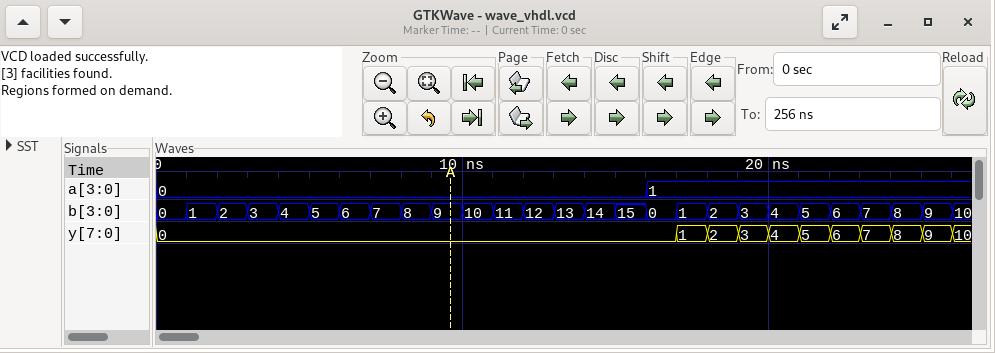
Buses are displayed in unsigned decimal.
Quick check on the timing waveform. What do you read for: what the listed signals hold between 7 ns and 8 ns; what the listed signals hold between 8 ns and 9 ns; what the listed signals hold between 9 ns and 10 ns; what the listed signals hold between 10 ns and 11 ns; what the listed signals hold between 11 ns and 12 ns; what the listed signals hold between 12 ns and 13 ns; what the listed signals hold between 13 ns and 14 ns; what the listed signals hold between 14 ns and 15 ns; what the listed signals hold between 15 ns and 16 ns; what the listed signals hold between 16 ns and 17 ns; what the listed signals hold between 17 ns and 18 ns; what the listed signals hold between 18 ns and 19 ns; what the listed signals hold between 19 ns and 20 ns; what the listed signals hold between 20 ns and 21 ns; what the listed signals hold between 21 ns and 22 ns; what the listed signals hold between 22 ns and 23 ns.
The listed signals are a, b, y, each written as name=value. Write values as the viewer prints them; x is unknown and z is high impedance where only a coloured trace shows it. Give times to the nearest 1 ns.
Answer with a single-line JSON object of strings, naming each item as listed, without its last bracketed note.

{"what the listed signals hold between 7 ns and 8 ns": "a=0, b=7, y=0", "what the listed signals hold between 8 ns and 9 ns": "a=0, b=8, y=0", "what the listed signals hold between 9 ns and 10 ns": "a=0, b=9, y=0", "what the listed signals hold between 10 ns and 11 ns": "a=0, b=10, y=0", "what the listed signals hold between 11 ns and 12 ns": "a=0, b=11, y=0", "what the listed signals hold between 12 ns and 13 ns": "a=0, b=12, y=0", "what the listed signals hold between 13 ns and 14 ns": "a=0, b=13, y=0", "what the listed signals hold between 14 ns and 15 ns": "a=0, b=14, y=0", "what the listed signals hold between 15 ns and 16 ns": "a=0, b=15, y=0", "what the listed signals hold between 16 ns and 17 ns": "a=1, b=0, y=0", "what the listed signals hold between 17 ns and 18 ns": "a=1, b=1, y=1", "what the listed signals hold between 18 ns and 19 ns": "a=1, b=2, y=2", "what the listed signals hold between 19 ns and 20 ns": "a=1, b=3, y=3", "what the listed signals hold between 20 ns and 21 ns": "a=1, b=4, y=4", "what the listed signals hold between 21 ns and 22 ns": "a=1, b=5, y=5", "what the listed signals hold between 22 ns and 23 ns": "a=1, b=6, y=6"}
